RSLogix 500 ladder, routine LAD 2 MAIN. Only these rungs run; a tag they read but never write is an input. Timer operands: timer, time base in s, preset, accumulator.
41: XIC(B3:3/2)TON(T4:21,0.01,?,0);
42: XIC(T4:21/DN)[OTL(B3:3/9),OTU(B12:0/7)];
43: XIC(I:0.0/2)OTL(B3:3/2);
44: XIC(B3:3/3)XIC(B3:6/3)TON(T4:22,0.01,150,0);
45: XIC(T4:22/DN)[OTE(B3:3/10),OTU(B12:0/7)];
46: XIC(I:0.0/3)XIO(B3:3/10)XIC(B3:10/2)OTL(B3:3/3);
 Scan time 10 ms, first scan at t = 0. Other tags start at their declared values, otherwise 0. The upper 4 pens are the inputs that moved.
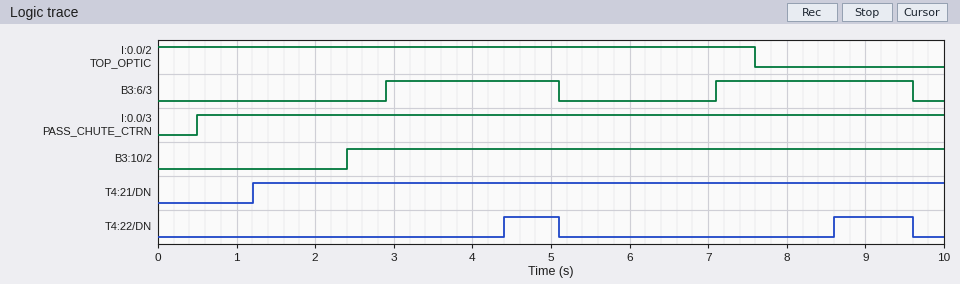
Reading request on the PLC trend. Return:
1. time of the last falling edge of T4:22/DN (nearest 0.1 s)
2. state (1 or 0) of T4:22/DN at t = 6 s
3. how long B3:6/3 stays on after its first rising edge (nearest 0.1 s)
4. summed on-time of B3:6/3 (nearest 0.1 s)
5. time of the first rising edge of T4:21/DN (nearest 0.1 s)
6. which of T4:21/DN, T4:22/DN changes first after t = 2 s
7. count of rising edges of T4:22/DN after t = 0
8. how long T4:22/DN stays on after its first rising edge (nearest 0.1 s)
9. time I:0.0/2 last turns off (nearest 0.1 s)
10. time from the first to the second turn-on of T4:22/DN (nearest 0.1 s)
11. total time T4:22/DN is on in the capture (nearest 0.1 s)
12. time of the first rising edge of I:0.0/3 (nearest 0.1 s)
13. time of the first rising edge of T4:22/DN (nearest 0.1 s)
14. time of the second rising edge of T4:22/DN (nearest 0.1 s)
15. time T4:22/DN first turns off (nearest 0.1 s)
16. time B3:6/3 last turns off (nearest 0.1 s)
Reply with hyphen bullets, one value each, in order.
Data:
- 9.6 s
- 0
- 2.2 s
- 4.7 s
- 1.2 s
- T4:22/DN
- 2
- 0.7 s
- 7.6 s
- 4.2 s
- 1.7 s
- 0.5 s
- 4.4 s
- 8.6 s
- 5.1 s
- 9.6 s
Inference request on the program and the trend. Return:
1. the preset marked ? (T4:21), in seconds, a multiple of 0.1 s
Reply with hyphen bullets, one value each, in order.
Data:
- 1.2 s
